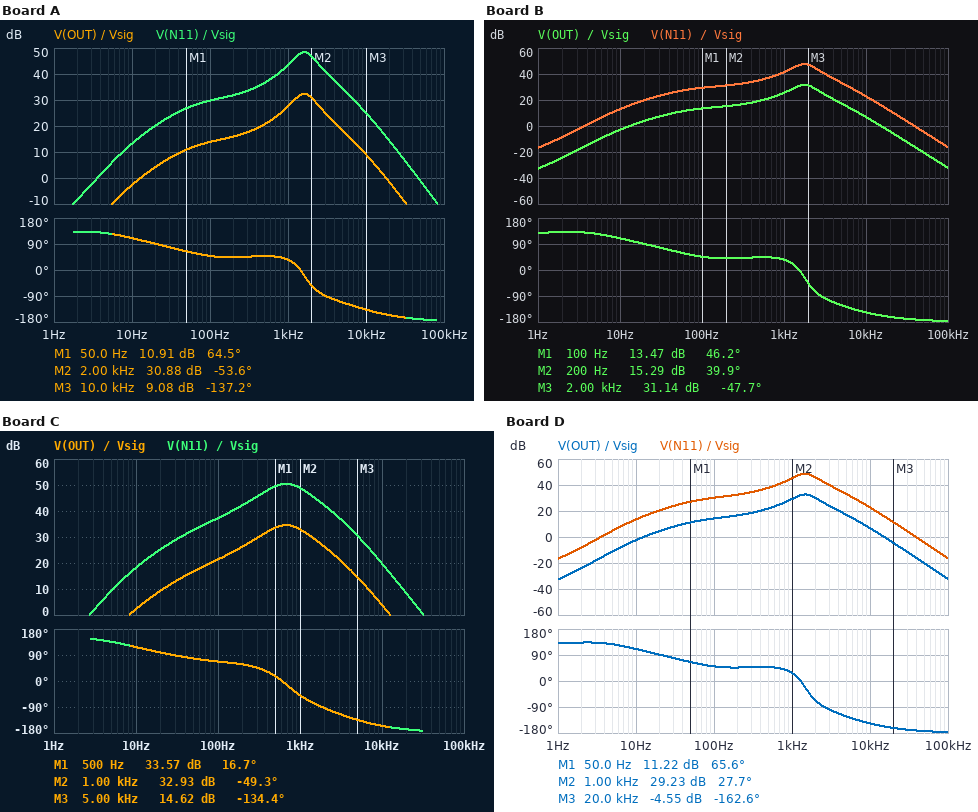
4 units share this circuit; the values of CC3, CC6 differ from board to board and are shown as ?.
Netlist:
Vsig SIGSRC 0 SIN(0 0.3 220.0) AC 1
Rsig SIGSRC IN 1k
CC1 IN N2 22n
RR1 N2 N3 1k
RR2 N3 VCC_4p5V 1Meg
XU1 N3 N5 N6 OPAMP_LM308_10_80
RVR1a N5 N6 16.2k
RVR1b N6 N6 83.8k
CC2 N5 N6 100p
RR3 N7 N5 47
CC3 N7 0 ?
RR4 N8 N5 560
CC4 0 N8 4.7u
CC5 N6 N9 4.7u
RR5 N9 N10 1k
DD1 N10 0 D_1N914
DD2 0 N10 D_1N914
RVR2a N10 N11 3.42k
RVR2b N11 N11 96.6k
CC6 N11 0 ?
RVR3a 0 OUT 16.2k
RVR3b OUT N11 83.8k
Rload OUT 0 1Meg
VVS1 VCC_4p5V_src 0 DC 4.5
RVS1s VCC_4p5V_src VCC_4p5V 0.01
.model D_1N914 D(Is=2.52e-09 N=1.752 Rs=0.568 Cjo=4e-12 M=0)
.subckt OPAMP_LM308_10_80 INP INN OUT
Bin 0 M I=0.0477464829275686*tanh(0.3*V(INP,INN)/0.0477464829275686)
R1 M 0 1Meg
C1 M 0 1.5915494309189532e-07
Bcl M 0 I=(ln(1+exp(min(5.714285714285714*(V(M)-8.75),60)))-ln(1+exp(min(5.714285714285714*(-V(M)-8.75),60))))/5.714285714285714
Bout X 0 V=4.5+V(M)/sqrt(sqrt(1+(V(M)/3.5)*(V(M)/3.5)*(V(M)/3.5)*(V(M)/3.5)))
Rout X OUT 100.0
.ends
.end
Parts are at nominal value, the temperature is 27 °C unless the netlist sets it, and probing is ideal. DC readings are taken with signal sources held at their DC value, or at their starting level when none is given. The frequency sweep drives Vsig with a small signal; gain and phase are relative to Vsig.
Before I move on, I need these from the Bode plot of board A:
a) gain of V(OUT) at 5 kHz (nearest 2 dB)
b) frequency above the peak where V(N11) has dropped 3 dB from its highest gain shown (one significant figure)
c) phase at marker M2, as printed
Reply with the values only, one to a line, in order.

18 dB
2 kHz
-53.6 deg
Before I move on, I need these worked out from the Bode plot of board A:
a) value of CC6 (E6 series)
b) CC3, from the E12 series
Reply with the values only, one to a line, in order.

4.7 nF
1 µF
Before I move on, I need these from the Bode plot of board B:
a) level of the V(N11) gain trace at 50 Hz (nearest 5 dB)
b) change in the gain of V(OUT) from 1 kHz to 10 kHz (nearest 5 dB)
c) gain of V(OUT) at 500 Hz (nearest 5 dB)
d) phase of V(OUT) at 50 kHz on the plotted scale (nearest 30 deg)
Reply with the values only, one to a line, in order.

25 dB
-20 dB
20 dB
-180 deg
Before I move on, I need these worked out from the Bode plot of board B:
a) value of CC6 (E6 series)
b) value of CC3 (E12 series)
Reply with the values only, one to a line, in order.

6.8 nF
820 nF
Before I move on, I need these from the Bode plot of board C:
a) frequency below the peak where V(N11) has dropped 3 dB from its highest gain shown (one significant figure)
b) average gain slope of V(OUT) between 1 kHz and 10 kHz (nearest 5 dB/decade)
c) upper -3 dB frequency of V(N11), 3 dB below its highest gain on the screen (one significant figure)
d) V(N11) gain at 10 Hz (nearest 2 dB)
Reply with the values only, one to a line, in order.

400 Hz
-30 dB/decade
1 kHz
18 dB
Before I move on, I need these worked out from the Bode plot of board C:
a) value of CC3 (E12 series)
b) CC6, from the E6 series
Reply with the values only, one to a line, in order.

5.6 µF
10 nF
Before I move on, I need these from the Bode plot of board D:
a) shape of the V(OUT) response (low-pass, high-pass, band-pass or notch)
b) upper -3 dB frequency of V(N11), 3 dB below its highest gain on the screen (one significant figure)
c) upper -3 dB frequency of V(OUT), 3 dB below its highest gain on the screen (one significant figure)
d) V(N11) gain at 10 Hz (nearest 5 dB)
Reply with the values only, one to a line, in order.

band-pass
2 kHz
2 kHz
15 dB
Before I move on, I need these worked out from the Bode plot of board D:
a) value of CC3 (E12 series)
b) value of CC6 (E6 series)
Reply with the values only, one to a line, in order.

1.2 µF
6.8 nF
